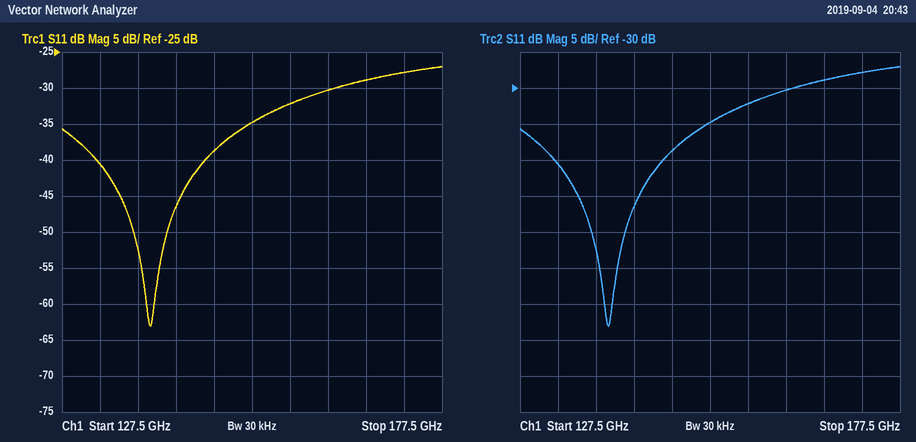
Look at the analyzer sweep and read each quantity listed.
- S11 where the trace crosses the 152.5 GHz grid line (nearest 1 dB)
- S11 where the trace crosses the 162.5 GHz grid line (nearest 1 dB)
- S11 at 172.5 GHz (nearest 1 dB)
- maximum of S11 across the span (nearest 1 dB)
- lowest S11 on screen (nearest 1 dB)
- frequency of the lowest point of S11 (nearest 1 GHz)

-35 dB
-30 dB
-28 dB
-27 dB
-63 dB
139 GHz
